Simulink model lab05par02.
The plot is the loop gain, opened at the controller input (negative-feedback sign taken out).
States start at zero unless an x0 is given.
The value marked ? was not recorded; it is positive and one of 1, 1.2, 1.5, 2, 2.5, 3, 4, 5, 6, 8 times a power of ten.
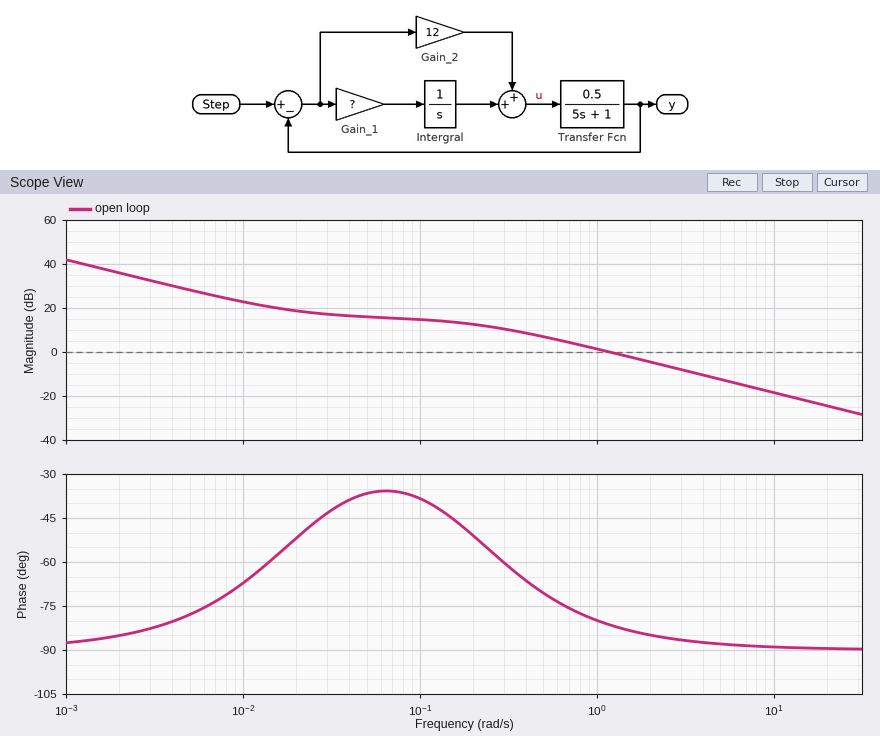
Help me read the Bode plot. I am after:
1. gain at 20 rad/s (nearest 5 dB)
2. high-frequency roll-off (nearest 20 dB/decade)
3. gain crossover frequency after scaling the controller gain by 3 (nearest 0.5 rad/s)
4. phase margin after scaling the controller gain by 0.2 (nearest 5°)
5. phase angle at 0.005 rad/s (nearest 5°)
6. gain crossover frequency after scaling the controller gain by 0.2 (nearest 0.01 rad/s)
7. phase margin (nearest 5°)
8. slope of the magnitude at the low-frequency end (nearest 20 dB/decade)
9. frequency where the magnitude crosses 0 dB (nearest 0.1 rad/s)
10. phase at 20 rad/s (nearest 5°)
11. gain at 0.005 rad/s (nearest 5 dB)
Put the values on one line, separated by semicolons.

-25 dB; -20 dB/decade; 3.5 rad/s; 135°; -80°; 0.14 rad/s; 100°; -20 dB/decade; 1.2 rad/s; -90°; 30 dB
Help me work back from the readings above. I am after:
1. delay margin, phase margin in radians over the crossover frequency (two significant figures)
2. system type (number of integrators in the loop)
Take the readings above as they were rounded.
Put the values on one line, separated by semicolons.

1.5 s; 1
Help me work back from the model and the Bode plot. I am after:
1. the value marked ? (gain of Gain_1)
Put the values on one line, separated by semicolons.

0.25
